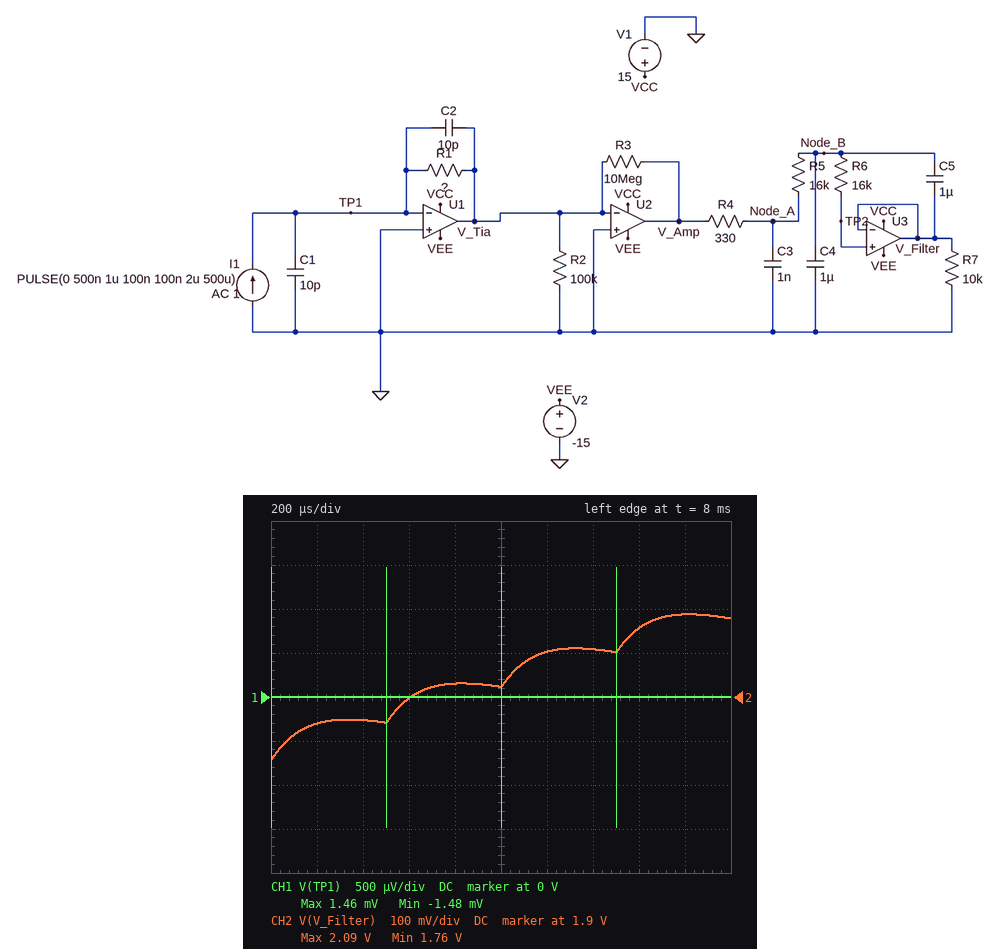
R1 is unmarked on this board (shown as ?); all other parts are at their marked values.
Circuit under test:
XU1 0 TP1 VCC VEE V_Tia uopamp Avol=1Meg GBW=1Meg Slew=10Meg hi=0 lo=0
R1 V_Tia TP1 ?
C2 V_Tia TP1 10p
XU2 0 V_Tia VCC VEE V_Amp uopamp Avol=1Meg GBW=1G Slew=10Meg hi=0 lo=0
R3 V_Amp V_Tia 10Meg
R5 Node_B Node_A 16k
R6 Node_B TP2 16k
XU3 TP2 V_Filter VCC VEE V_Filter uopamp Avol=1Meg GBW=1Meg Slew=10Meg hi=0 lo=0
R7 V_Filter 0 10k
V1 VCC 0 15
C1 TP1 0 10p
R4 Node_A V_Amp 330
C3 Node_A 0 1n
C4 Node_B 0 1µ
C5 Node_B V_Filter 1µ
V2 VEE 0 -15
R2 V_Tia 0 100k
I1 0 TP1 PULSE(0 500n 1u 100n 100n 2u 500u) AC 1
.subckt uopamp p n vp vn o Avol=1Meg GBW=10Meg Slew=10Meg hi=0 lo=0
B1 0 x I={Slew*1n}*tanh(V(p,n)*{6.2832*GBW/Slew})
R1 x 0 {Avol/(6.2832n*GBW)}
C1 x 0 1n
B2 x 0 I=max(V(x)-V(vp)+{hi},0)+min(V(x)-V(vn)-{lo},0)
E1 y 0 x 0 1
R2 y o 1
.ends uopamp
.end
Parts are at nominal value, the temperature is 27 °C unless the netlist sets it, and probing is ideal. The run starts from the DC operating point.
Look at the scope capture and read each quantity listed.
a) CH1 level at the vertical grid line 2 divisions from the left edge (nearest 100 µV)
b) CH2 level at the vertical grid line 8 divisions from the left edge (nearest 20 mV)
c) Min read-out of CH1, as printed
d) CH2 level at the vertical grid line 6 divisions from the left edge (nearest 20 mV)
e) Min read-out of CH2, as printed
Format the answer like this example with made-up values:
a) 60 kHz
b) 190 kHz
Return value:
a) 0 V
b) 2.06 V
c) -1.48 mV
d) 2.00 V
e) 1.76 V
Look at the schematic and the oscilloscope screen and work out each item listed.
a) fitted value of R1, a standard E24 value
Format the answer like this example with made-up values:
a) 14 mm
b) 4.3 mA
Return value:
a) 6.2 kΩ
